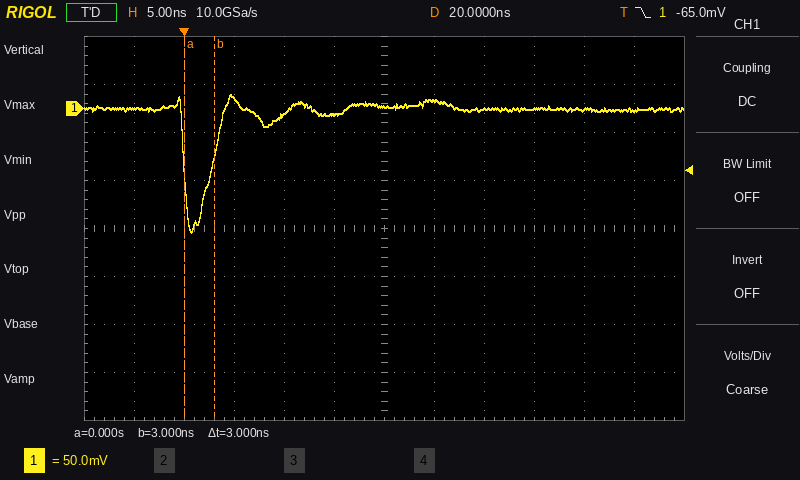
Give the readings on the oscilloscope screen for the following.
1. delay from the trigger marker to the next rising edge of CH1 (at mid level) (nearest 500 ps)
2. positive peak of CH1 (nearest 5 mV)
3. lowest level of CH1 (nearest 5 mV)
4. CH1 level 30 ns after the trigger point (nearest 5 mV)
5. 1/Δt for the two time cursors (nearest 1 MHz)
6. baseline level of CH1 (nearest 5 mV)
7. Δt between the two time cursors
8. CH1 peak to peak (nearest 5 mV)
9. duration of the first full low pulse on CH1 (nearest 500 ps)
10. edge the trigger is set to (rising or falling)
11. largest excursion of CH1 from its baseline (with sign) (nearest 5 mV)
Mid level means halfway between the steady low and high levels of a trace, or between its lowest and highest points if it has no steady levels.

3.0 ns
15 mV
-130 mV
0 mV
333 MHz
0 mV
3 ns
145 mV
3.0 ns
falling
-130 mV
